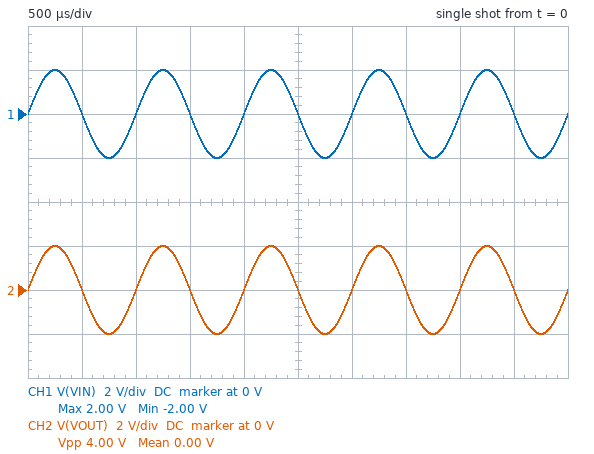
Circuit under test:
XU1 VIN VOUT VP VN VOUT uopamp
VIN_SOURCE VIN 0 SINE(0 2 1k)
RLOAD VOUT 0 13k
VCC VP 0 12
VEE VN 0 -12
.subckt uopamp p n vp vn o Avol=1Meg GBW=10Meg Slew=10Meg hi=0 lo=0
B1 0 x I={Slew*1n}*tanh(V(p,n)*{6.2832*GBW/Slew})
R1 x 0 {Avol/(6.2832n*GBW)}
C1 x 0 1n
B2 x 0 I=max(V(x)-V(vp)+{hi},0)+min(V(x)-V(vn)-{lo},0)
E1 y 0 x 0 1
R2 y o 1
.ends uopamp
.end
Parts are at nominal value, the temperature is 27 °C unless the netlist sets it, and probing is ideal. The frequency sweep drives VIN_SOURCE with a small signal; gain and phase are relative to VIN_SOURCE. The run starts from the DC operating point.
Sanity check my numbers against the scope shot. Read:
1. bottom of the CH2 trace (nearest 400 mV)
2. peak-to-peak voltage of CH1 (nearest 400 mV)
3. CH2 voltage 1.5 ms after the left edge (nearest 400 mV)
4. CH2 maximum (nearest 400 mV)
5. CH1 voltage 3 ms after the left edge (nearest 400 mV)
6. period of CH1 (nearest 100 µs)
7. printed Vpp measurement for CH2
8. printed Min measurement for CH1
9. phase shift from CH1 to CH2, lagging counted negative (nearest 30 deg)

-2.0 V
4.0 V
0 V
2.0 V
0 V
1.0 ms
4.00 V
-2.00 V
0 deg
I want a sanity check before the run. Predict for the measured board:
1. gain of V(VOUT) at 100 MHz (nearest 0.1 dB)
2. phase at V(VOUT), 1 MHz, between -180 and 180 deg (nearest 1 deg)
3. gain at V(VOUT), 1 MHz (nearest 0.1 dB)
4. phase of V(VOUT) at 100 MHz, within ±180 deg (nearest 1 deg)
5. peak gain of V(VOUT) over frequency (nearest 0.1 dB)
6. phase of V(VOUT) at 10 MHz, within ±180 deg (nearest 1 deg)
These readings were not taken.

-20.0 dB
-6 deg
0 dB
-84 deg
0 dB
-45 deg
